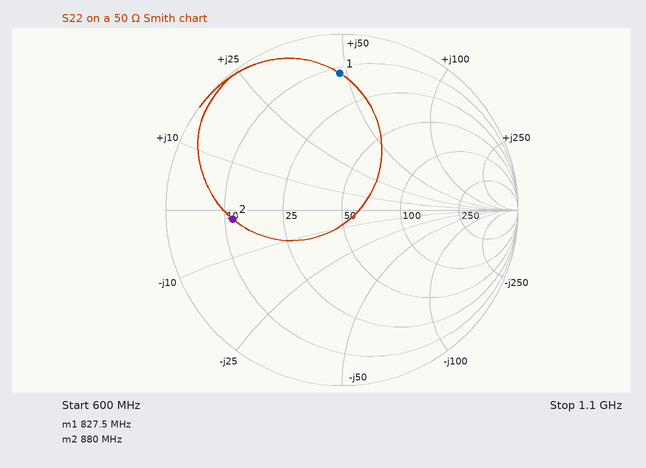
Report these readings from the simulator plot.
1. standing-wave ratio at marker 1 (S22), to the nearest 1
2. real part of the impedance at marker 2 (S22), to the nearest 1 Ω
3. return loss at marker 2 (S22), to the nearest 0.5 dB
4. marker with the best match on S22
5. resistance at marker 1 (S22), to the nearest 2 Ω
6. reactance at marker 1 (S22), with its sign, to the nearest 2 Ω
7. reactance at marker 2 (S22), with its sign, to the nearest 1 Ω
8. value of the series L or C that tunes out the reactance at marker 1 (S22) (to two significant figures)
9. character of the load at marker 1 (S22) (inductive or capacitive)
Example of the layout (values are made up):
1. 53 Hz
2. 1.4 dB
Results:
1. 8
2. 12 Ω
3. 4.0 dB
4. marker 2
5. 12 Ω
6. +48 Ω
7. -2 Ω
8. 4.0 pF
9. inductive
